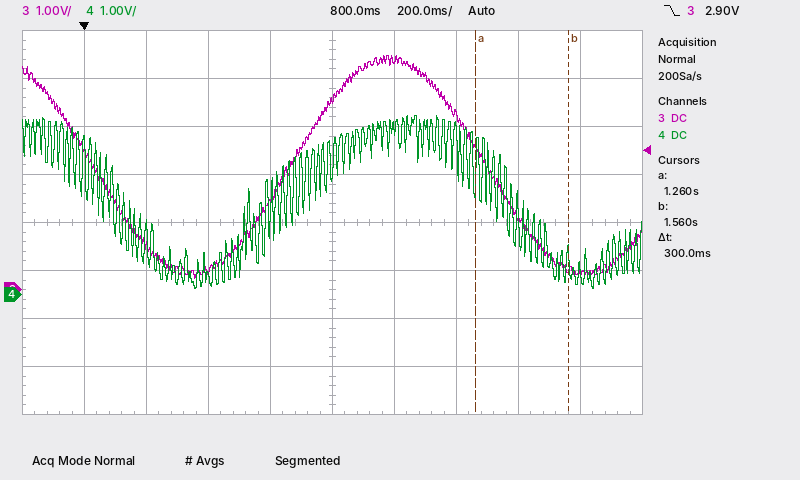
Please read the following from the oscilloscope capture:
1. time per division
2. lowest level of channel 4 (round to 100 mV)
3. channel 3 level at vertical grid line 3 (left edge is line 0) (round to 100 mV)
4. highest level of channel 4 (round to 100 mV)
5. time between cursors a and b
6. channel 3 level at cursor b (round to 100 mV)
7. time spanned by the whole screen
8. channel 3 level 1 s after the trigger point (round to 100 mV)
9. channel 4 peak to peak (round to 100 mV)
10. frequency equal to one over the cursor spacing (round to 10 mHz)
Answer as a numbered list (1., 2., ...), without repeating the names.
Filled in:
1. 200 ms
2. 100 mV
3. 400 mV
4. 3.7 V
5. 300 ms
6. 400 mV
7. 2 s
8. 4.8 V
9. 3.6 V
10. 3.33 Hz
